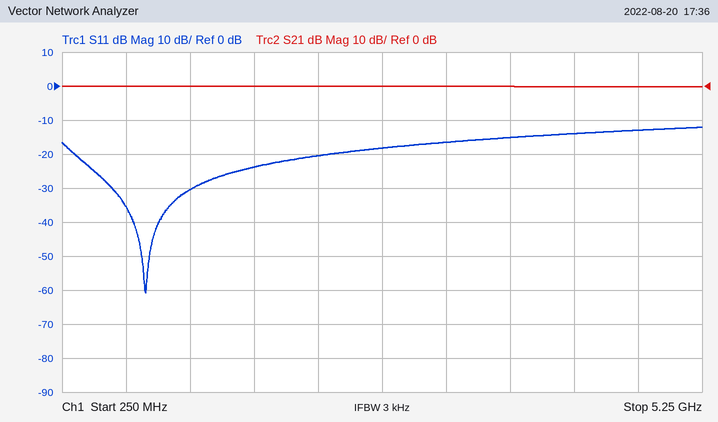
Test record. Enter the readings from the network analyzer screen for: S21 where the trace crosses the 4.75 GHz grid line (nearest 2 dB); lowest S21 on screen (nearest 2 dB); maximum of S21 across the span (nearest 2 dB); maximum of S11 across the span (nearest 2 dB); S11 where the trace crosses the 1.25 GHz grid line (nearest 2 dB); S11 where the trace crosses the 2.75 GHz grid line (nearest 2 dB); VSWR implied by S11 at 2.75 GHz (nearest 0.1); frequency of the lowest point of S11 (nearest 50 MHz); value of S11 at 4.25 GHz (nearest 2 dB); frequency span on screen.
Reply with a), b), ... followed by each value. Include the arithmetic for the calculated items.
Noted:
a) 0 dB
b) 0 dB
c) 0 dB
d) -12 dB
e) -30 dB
f) -18 dB
g) |Γ| = 10^(-18/20) = 0.1259; VSWR = (1 + 0.1259)/(1 − 0.1259) ≈ 1.3
h) 900 MHz
i) -14 dB
j) 5 GHz
